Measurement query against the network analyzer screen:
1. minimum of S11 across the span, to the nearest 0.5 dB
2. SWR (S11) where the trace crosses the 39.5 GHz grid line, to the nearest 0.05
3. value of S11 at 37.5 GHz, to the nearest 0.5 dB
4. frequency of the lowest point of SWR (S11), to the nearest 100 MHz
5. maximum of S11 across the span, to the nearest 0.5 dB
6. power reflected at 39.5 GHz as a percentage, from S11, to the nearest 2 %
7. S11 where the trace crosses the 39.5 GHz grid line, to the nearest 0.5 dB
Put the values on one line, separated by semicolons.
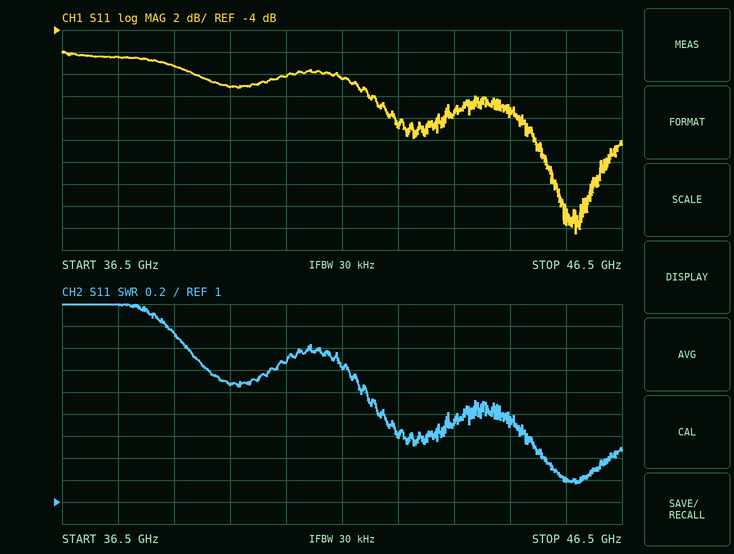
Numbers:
-22.5 dB; 2.05; -6.5 dB; 45.7 GHz; -6.0 dB; 12 %; -9.0 dB
